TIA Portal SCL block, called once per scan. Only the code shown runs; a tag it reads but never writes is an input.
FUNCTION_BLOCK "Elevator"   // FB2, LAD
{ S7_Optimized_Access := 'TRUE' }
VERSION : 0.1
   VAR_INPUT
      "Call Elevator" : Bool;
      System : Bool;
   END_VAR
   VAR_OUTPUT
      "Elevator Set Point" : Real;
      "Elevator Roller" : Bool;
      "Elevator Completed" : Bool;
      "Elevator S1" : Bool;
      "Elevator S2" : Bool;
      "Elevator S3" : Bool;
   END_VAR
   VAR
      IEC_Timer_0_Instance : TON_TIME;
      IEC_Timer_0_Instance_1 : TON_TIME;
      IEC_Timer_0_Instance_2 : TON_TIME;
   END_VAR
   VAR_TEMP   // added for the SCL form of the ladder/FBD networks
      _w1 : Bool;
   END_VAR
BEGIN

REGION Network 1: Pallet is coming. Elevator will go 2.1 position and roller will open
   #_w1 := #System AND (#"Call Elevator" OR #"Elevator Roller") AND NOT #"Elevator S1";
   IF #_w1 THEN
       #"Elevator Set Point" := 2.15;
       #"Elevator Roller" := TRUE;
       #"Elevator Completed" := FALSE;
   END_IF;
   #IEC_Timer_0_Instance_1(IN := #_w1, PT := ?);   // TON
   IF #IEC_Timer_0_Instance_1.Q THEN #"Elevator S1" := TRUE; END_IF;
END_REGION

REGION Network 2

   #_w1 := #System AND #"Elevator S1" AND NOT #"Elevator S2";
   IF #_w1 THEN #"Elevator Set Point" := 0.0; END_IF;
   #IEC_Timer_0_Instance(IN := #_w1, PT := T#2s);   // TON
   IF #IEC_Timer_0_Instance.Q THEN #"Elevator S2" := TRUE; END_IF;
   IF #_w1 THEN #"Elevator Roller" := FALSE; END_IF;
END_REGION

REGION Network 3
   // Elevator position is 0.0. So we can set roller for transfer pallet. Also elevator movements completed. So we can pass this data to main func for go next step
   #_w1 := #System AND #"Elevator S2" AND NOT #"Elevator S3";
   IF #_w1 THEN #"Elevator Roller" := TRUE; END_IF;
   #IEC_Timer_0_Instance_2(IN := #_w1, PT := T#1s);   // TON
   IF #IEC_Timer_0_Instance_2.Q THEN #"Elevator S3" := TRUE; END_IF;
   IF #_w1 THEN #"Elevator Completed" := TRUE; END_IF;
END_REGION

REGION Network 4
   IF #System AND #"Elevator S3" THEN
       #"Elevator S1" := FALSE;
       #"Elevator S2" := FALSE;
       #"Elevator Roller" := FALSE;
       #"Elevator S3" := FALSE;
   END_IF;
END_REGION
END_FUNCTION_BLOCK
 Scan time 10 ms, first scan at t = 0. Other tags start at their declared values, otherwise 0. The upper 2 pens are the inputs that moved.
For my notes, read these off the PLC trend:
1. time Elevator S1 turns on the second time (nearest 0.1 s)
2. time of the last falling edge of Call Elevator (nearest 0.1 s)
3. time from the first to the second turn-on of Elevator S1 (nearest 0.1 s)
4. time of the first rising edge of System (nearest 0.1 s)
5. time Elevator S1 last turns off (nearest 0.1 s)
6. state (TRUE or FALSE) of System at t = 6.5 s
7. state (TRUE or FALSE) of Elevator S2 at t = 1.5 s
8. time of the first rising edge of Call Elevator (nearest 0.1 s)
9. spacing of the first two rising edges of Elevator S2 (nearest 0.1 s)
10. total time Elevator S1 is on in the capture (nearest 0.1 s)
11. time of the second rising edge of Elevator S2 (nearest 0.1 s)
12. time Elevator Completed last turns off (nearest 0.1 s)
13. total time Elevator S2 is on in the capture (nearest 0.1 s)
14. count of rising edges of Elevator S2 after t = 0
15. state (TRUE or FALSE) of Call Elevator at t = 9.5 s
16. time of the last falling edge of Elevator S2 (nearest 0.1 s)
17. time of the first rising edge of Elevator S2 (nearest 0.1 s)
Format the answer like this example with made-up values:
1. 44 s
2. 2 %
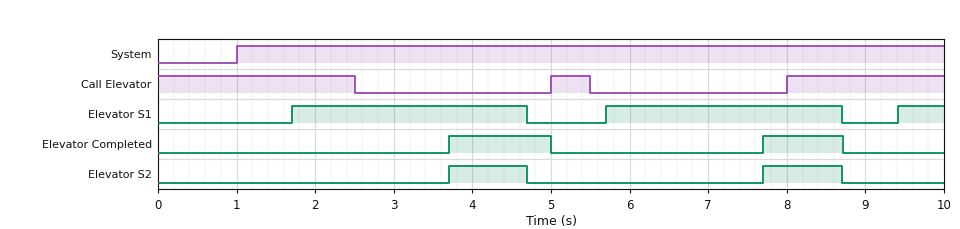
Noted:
1. 5.7 s
2. 5.5 s
3. 4.0 s
4. 1.0 s
5. 8.7 s
6. TRUE
7. FALSE
8. 5.0 s
9. 4.0 s
10. 6.6 s
11. 7.7 s
12. 8.7 s
13. 2.0 s
14. 2
15. TRUE
16. 8.7 s
17. 3.7 s
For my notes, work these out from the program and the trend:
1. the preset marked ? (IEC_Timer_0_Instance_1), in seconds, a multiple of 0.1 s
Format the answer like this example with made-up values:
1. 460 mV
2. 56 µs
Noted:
1. 0.7 s
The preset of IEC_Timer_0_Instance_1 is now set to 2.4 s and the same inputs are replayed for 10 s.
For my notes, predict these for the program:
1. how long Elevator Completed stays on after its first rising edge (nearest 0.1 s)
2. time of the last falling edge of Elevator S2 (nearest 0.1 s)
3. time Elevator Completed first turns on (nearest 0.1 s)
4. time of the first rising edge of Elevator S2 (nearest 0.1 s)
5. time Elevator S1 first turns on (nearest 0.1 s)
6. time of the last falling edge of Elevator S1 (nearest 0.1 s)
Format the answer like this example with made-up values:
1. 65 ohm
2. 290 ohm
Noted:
1. 2.6 s
2. 6.4 s
3. 5.4 s
4. 5.4 s
5. 3.4 s
6. 6.4 s
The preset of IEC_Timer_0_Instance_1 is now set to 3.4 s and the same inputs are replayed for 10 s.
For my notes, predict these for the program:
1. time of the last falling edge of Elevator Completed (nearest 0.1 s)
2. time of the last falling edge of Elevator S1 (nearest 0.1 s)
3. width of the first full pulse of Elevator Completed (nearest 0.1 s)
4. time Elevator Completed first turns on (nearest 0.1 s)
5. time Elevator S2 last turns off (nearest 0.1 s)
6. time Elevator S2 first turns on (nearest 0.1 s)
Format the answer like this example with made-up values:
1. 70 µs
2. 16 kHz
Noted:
1. 8.0 s
2. 7.4 s
3. 1.6 s
4. 6.4 s
5. 7.4 s
6. 6.4 s
